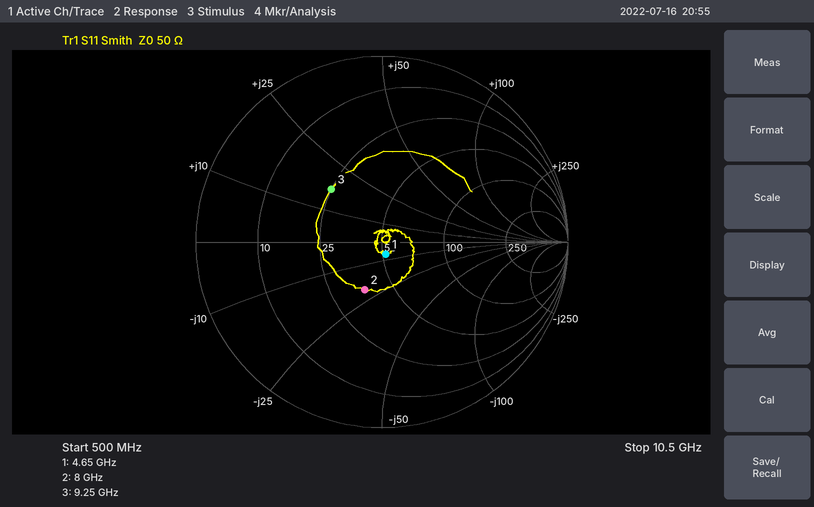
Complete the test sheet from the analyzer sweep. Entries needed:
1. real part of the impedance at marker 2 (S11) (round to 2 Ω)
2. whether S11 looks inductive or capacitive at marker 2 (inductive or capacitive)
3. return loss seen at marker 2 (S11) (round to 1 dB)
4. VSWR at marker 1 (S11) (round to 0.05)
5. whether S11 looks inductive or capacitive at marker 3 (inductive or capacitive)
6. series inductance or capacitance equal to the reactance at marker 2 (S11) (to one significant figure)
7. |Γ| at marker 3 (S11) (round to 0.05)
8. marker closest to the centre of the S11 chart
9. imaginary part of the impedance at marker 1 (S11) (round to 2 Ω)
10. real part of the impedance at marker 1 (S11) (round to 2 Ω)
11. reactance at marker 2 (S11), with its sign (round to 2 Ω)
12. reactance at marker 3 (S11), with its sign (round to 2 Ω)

36 Ω
capacitive
11 dB
1.15
inductive
1.0 pF
0.40
marker 1
-6 Ω
52 Ω
-20 Ω
+16 Ω
